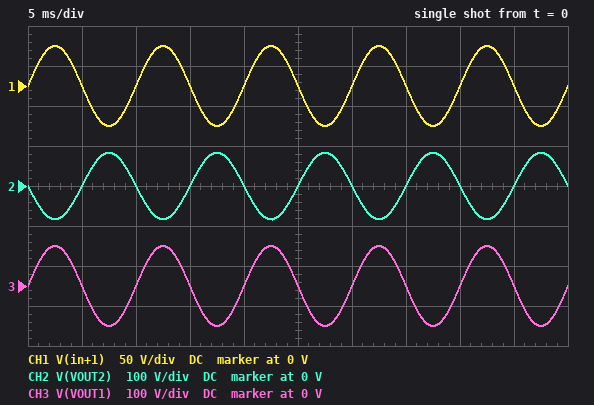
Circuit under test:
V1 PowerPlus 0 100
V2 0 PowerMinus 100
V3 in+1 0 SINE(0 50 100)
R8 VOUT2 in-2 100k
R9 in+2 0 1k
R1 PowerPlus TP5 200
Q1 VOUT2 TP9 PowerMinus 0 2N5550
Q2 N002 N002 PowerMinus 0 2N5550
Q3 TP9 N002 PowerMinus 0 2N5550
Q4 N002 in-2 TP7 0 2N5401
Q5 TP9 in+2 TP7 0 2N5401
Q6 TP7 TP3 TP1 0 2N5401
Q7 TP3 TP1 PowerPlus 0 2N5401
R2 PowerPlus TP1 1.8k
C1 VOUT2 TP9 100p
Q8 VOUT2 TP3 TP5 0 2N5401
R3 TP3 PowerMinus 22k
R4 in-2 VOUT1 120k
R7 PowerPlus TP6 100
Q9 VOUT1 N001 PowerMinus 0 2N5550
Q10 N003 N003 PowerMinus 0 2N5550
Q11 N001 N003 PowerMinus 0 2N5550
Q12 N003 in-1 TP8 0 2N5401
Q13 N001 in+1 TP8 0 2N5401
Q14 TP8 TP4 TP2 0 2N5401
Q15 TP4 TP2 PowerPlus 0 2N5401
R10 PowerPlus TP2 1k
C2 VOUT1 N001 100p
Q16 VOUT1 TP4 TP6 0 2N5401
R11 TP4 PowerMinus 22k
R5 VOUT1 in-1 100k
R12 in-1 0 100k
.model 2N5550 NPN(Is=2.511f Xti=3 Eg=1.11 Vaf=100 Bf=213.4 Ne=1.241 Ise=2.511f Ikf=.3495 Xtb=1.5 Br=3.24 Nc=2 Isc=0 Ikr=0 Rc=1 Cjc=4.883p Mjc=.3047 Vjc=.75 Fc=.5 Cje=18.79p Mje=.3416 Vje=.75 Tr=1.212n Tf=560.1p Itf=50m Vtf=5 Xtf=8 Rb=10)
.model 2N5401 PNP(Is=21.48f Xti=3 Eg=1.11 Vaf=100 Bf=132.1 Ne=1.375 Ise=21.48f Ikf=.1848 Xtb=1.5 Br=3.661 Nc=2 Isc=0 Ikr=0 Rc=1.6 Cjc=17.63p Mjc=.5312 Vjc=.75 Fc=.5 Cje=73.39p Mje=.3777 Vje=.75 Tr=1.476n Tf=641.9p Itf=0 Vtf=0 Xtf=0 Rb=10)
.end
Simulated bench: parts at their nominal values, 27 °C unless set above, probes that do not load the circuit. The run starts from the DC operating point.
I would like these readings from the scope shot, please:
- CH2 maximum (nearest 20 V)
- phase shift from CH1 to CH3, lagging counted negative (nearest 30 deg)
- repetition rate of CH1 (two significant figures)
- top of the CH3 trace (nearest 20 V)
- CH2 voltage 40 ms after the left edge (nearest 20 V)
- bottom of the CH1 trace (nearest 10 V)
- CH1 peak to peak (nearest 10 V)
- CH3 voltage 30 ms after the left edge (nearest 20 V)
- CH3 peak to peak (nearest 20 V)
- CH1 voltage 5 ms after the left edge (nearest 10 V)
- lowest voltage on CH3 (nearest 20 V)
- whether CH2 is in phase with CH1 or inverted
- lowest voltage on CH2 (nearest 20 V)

80 V
0 deg
100 Hz
100 V
0 V
-50 V
100 V
0 V
200 V
0 V
-100 V
inverted
-80 V
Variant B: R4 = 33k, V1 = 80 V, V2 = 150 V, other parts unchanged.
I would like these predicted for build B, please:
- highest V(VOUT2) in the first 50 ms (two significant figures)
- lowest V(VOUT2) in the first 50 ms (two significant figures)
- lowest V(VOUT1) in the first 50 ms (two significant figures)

79 V
-150 V
-100 V
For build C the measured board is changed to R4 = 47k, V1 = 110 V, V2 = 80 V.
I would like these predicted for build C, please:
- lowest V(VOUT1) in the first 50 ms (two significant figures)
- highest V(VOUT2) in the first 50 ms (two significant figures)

-80 V
110 V
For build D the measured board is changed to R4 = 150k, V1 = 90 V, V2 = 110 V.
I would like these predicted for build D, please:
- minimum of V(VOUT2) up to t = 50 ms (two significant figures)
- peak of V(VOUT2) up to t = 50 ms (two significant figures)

-60 V
67 V
